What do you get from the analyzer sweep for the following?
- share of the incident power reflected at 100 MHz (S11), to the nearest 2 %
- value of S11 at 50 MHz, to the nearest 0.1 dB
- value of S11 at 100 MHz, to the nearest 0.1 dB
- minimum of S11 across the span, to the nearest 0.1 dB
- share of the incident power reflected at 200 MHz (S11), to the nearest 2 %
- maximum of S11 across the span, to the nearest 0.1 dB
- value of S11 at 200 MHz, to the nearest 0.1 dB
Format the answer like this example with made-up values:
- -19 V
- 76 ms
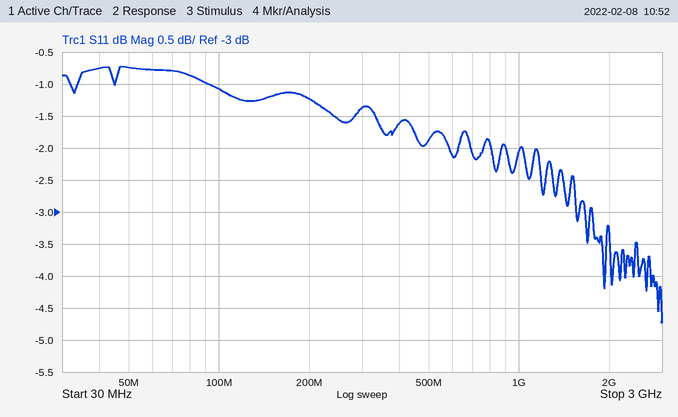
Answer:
- 78 %
- -0.7 dB
- -1.1 dB
- -4.7 dB
- 76 %
- -0.7 dB
- -1.2 dB
